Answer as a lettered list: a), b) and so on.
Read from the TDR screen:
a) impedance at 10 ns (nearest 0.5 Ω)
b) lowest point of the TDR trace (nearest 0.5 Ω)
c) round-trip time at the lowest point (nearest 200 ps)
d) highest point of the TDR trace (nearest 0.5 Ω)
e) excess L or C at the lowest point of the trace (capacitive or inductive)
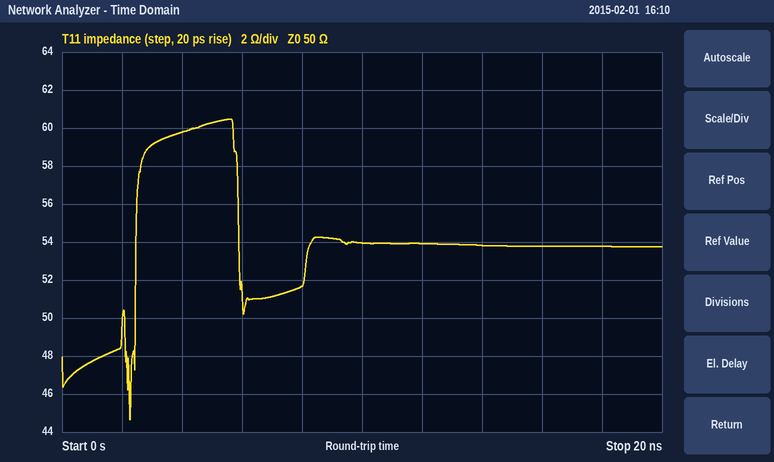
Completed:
a) 54.0 Ω
b) 44.5 Ω
c) 2.2 ns
d) 60.5 Ω
e) capacitive
